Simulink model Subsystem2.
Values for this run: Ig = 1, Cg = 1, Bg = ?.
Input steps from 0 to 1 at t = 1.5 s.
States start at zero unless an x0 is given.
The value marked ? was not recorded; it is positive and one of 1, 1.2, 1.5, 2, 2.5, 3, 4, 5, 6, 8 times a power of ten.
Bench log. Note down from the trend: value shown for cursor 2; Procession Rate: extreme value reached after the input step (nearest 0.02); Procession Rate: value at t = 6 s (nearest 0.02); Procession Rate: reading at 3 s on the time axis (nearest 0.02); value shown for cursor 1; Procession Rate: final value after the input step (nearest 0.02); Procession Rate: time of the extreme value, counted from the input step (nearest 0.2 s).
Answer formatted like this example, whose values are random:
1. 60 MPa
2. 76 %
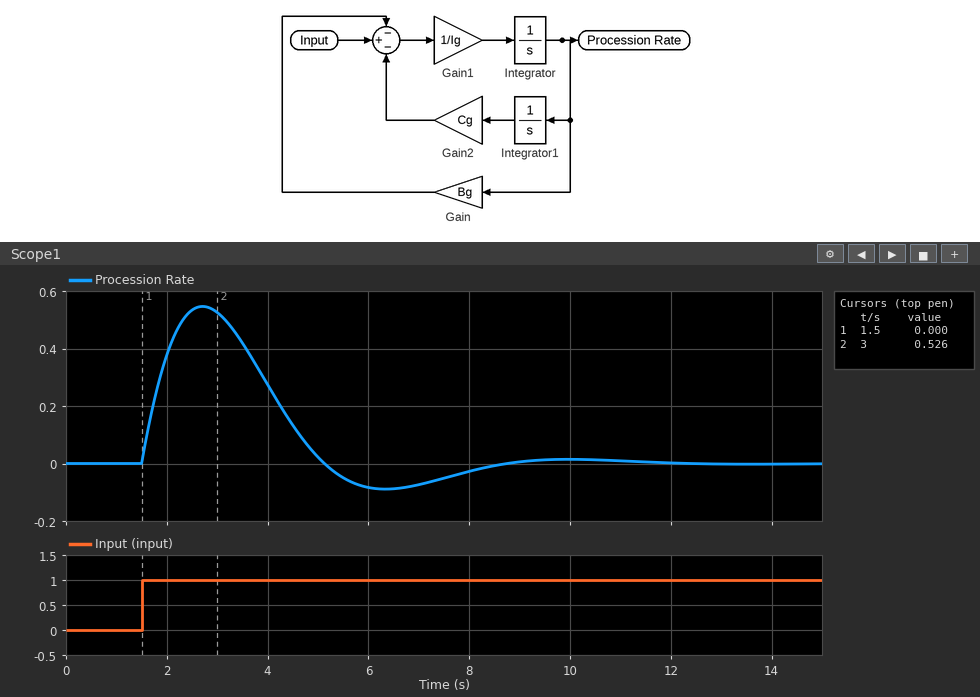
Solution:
1. 0.526
2. 0.54
3. -0.08
4. 0.52
5. 0.000
6. 0.00
7. 1.2 s
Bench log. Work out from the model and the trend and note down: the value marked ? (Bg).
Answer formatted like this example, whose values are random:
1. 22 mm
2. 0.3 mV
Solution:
1. 1
